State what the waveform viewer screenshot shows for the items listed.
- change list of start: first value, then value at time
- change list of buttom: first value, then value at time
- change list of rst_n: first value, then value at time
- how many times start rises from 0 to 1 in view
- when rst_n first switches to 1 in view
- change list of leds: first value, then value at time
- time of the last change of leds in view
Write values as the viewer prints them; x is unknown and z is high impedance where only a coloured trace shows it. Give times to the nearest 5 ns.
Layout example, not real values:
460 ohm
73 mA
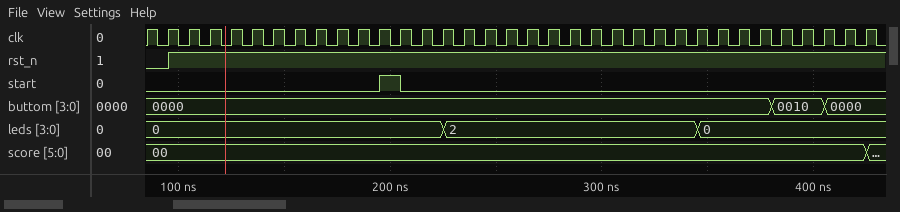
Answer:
0, 1 at 195 ns, 0 at 205 ns
0000, 0010 at 380 ns, 0000 at 405 ns
0, 1 at 95 ns
1
95 ns
0, 2 at 225 ns, 0 at 345 ns
345 ns
